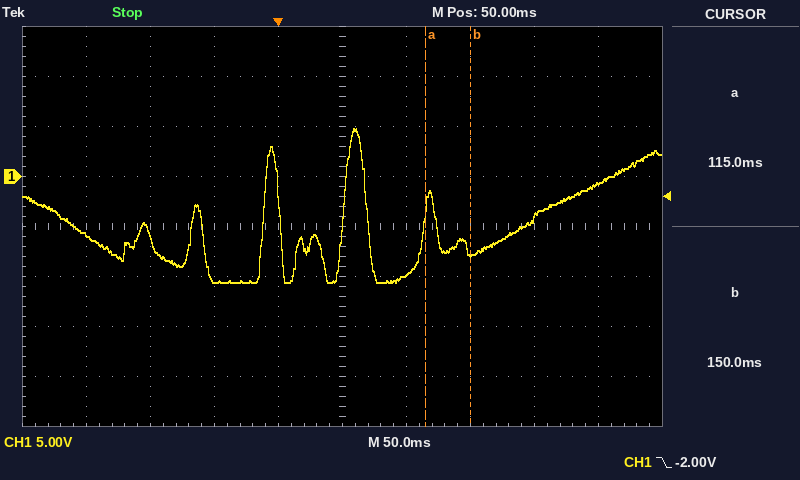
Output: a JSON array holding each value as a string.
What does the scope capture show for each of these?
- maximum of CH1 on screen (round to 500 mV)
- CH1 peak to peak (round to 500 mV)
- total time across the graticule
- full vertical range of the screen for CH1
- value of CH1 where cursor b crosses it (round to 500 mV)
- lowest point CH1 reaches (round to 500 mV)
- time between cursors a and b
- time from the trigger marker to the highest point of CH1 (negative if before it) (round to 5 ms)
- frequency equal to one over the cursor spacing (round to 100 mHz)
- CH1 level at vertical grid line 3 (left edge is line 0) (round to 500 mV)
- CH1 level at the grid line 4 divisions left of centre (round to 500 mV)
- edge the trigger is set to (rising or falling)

["5.0 V", "15.5 V", "500 ms", "40 V", "-7.5 V", "-10.5 V", "35 ms", "+60 ms", "28.6 Hz", "-10.5 V", "-6.0 V", "falling"]
